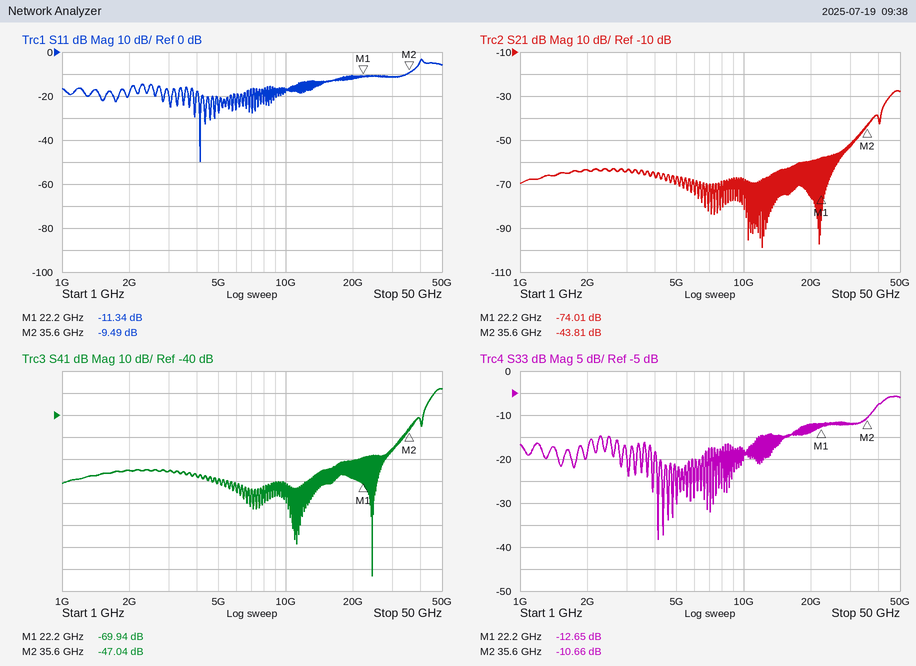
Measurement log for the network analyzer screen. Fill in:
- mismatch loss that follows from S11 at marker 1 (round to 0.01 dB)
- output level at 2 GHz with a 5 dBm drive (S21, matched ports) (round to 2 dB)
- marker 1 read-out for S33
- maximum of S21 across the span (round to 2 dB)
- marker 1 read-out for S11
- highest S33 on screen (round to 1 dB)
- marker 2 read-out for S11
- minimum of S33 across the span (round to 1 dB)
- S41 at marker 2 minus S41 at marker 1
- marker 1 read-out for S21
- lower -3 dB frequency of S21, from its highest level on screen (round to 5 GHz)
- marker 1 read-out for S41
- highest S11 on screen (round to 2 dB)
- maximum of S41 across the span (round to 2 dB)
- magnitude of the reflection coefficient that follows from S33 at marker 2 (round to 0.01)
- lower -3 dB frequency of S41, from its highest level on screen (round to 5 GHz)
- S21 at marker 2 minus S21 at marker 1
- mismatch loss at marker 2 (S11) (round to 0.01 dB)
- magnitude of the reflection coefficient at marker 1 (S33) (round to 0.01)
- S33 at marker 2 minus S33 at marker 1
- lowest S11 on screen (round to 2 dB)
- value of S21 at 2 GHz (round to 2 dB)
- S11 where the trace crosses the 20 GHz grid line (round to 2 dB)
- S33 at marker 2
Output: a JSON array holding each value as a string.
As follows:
["0.33 dB", "-58 dBm", "-12.65 dB", "-28 dB", "-11.34 dB", "-6 dB", "-9.49 dB", "-38 dB", "22.90 dB", "-74.01 dB", "45 GHz", "-69.94 dB", "-4 dB", "-28 dB", "0.29", "45 GHz", "30.20 dB", "0.52 dB", "0.23", "1.99 dB", "-50 dB", "-64 dB", "-12 dB", "-10.66 dB"]
